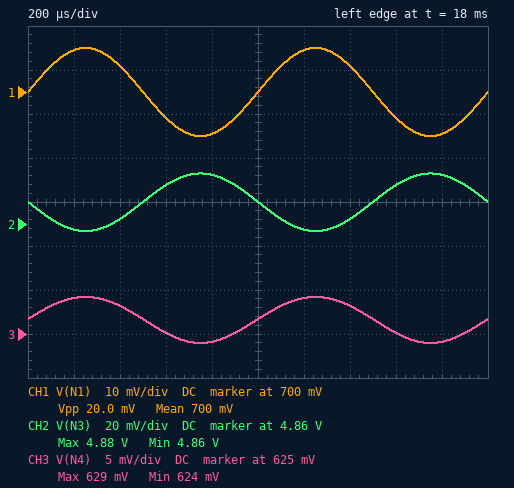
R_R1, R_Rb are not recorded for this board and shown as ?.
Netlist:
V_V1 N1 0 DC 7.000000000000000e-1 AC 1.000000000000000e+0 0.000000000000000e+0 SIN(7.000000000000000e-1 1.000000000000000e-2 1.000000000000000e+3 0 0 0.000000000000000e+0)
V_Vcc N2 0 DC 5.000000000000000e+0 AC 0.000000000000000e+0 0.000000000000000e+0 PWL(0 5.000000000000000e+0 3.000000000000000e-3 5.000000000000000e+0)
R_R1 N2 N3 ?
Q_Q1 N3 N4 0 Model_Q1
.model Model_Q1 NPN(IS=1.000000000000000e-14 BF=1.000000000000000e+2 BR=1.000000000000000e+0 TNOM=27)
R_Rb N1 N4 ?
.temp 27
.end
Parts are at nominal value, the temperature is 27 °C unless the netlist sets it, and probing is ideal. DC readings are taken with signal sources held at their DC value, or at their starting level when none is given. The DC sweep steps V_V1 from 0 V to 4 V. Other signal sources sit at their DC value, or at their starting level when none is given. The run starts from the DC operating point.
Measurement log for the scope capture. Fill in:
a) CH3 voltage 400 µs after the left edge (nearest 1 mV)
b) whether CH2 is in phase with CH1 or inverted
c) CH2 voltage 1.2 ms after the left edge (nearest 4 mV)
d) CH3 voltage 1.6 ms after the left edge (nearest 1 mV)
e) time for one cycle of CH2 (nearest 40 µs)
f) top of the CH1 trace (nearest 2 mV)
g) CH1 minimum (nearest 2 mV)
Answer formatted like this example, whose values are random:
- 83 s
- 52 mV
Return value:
- 628 mV
- inverted
- 4.856 V
- 625 mV
- 1.00 ms
- 710 mV
- 690 mV
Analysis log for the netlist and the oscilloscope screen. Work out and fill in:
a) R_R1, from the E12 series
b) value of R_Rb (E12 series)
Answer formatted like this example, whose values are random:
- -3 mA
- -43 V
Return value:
- 390 Ω
- 22 kΩ
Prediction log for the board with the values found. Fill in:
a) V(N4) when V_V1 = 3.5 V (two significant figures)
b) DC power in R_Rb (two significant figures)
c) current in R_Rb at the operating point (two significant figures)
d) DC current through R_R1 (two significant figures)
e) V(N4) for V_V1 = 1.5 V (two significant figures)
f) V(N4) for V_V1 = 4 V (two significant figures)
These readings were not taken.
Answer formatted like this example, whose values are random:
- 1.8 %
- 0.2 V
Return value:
- 720 mV
- 240 nW
- 3.3 µA
- 330 µA
- 690 mV
- 720 mV
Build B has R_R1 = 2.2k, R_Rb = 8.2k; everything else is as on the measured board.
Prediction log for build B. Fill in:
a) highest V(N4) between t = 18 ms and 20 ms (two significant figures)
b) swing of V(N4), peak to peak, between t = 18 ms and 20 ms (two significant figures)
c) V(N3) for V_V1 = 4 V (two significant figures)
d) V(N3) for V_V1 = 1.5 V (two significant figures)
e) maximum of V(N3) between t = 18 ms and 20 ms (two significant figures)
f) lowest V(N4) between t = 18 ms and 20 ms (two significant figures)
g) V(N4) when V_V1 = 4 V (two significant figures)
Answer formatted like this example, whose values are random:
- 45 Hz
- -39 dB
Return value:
- 650 mV
- 6.4 mV
- 54 mV
- 89 mV
- 3.7 V
- 640 mV
- 680 mV
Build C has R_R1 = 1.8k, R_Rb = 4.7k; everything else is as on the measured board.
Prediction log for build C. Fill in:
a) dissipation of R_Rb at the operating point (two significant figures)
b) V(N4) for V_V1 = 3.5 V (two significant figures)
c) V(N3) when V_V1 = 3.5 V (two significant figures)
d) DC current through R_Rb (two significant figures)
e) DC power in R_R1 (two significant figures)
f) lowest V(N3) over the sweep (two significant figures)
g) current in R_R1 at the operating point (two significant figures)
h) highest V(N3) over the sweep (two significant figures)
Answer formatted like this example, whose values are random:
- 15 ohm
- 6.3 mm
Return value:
- 440 nW
- 690 mV
- 50 mV
- 9.7 µA
- 1.7 mW
- 47 mV
- 970 µA
- 5.0 V
